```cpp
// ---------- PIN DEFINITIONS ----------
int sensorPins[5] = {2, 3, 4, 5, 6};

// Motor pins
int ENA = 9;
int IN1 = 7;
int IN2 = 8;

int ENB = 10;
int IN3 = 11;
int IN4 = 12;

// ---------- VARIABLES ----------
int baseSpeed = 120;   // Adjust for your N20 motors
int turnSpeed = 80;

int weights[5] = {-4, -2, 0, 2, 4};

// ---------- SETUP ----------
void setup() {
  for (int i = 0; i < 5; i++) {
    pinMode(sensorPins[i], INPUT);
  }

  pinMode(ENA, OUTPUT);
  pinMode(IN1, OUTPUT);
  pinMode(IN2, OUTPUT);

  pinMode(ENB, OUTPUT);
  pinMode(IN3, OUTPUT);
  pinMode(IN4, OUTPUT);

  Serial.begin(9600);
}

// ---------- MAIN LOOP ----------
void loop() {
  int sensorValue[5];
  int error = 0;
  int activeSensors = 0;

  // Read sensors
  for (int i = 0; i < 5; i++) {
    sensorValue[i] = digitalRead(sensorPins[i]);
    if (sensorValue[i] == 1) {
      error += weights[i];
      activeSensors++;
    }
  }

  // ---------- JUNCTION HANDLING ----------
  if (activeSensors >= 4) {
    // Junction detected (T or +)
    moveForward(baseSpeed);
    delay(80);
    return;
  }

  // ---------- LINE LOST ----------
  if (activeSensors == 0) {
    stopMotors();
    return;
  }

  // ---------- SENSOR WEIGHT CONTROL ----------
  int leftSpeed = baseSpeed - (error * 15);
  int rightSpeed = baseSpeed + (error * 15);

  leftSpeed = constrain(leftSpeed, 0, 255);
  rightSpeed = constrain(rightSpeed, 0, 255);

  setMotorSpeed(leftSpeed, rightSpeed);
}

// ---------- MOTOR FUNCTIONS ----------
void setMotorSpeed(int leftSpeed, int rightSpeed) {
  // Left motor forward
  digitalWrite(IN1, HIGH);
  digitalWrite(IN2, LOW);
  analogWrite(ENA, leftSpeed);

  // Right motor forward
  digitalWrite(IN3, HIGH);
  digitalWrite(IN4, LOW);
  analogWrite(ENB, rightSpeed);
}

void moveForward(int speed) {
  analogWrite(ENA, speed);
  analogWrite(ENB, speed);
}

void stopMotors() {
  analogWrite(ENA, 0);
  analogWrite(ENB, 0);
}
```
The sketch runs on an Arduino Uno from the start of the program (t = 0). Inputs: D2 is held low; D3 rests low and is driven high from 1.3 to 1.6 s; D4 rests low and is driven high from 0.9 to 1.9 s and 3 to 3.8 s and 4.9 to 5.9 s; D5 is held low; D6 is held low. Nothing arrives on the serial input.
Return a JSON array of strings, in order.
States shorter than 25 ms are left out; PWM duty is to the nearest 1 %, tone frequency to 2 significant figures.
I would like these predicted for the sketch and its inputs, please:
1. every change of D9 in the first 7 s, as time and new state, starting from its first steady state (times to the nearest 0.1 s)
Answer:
["0 s low; 0.9 s PWM 47 %; 1.3 s PWM 59 %; 1.6 s PWM 47 %; 1.9 s low; 3 s PWM 47 %; 3.8 s low; 4.9 s PWM 47 %; 5.9 s low"]
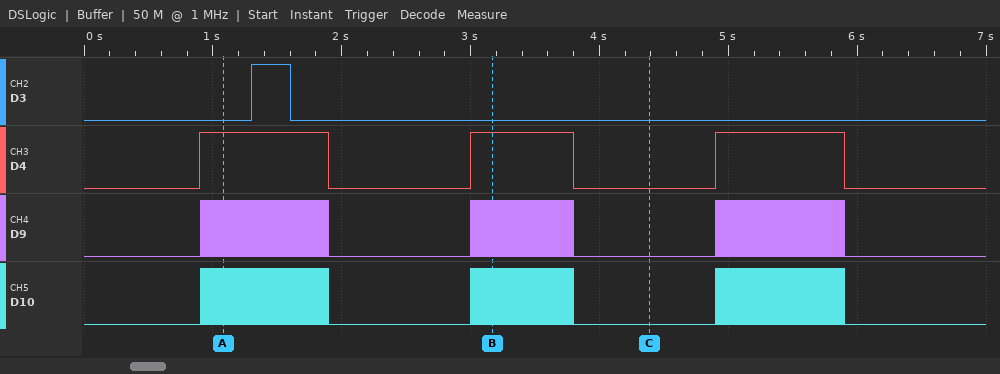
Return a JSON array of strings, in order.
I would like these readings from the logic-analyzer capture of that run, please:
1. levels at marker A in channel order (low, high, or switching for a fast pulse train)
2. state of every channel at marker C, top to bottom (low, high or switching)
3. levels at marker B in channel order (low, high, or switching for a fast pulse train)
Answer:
["D3 low, D4 high, D9 switching, D10 switching", "D3 low, D4 low, D9 low, D10 low", "D3 low, D4 high, D9 switching, D10 switching"]
